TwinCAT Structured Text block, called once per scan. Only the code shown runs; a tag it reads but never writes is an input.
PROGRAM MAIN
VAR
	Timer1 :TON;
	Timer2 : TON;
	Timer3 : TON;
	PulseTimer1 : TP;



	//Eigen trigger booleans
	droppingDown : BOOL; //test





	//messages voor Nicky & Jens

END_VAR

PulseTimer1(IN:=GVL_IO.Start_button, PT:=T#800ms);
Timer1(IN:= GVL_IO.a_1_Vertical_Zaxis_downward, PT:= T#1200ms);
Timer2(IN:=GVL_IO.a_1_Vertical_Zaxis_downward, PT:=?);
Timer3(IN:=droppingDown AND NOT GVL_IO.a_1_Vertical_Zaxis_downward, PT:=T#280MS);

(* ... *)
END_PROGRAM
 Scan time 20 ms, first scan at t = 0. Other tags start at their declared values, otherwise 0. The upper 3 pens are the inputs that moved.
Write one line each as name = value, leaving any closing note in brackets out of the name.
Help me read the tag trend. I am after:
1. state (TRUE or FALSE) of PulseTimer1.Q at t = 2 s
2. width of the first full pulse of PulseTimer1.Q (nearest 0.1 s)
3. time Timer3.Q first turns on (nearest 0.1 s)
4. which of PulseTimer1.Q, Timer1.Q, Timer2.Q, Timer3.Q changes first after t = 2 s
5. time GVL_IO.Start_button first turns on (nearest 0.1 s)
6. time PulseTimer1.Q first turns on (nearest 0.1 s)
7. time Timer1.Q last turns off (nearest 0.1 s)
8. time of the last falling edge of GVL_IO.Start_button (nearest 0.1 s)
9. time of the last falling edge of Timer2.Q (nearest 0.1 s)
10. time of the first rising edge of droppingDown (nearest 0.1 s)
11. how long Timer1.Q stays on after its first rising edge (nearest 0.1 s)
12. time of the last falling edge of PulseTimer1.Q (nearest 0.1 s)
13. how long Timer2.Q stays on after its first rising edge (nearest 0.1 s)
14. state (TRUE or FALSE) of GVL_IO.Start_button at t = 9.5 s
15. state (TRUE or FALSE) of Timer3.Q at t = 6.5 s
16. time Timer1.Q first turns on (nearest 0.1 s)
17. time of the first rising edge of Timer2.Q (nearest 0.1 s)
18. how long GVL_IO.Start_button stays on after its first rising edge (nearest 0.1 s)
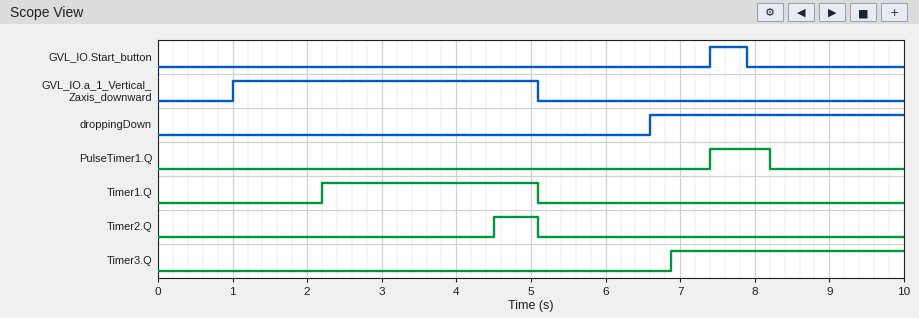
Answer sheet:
state (TRUE or FALSE) of PulseTimer1.Q at t = 2 s = FALSE
width of the first full pulse of PulseTimer1.Q = 0.8 s
time Timer3.Q first turns on = 6.9 s
which of PulseTimer1.Q, Timer1.Q, Timer2.Q, Timer3.Q changes first after t = 2 s = Timer1.Q
time GVL_IO.Start_button first turns on = 7.4 s
time PulseTimer1.Q first turns on = 7.4 s
time Timer1.Q last turns off = 5.1 s
time of the last falling edge of GVL_IO.Start_button = 7.9 s
time of the last falling edge of Timer2.Q = 5.1 s
time of the first rising edge of droppingDown = 6.6 s
how long Timer1.Q stays on after its first rising edge = 2.9 s
time of the last falling edge of PulseTimer1.Q = 8.2 s
how long Timer2.Q stays on after its first rising edge = 0.6 s
state (TRUE or FALSE) of GVL_IO.Start_button at t = 9.5 s = FALSE
state (TRUE or FALSE) of Timer3.Q at t = 6.5 s = FALSE
time Timer1.Q first turns on = 2.2 s
time of the first rising edge of Timer2.Q = 4.5 s
how long GVL_IO.Start_button stays on after its first rising edge = 0.5 s
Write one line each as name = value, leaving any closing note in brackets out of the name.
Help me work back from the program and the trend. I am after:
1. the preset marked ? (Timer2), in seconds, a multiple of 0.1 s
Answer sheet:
the preset marked ? (Timer2), in seconds, a multiple of 0.1 s = 3.5 s
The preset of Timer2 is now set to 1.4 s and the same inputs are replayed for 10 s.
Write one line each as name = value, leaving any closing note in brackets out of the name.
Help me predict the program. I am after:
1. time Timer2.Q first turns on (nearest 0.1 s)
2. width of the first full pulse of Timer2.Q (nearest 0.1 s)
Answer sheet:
time Timer2.Q first turns on = 2.4 s
width of the first full pulse of Timer2.Q = 2.7 s
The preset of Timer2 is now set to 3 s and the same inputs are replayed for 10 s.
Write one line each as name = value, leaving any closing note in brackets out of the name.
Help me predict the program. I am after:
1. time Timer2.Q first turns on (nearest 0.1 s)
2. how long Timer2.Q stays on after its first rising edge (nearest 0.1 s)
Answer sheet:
time Timer2.Q first turns on = 4.0 s
how long Timer2.Q stays on after its first rising edge = 1.1 s
